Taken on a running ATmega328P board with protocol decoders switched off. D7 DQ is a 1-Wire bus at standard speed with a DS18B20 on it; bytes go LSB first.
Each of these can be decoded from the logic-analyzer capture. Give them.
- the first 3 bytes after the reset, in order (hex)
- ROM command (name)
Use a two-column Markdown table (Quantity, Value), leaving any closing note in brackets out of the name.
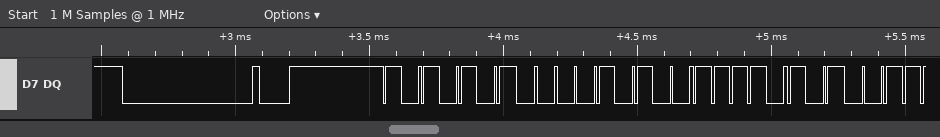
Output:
| Quantity | Value |
|---|---|
| the first 3 bytes after the reset, in order | 55 28 AF |
| ROM command | Match ROM |
